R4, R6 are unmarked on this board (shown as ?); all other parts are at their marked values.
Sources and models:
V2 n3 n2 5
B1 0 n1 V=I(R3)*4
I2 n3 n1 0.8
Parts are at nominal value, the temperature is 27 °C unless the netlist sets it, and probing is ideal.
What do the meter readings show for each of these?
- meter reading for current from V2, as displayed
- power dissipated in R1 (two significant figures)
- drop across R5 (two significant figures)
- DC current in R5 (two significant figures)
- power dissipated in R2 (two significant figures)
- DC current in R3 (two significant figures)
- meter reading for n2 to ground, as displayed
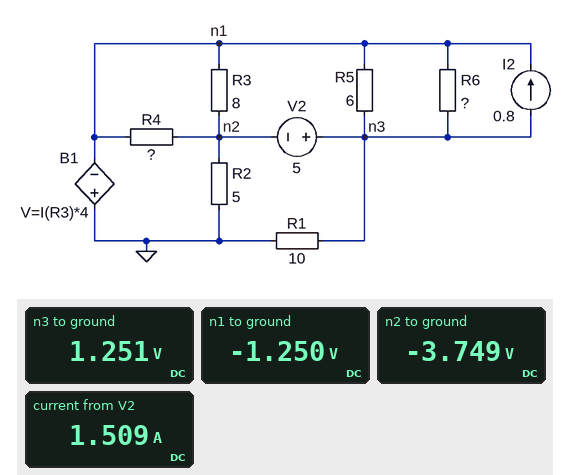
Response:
1.509 A
160 mW
2.5 V
420 mA
2.8 W
310 mA
-3.749 V
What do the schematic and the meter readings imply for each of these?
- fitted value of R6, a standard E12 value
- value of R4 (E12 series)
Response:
15 Ω
5.6 Ω
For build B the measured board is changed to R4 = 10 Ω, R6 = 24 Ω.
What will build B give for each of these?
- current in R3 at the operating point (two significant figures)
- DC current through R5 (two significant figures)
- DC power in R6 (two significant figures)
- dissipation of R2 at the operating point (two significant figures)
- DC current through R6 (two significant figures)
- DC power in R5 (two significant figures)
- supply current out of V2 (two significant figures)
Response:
330 mA
390 mA
230 mW
3.2 W
98 mA
920 mW
1.4 A
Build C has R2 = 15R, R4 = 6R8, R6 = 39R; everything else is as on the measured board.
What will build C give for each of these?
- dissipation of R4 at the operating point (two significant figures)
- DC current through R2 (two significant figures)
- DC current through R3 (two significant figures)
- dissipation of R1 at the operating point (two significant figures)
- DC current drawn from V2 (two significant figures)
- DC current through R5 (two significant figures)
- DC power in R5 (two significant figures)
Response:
1.5 W
320 mA
400 mA
6.3 mW
1.2 A
310 mA
560 mW
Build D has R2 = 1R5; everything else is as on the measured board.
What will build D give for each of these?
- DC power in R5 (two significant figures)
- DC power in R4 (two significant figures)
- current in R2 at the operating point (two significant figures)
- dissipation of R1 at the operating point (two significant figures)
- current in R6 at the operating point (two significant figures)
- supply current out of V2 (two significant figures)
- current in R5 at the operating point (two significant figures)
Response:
2.1 W
380 mW
1.5 A
790 mW
240 mA
1.9 A
590 mA
